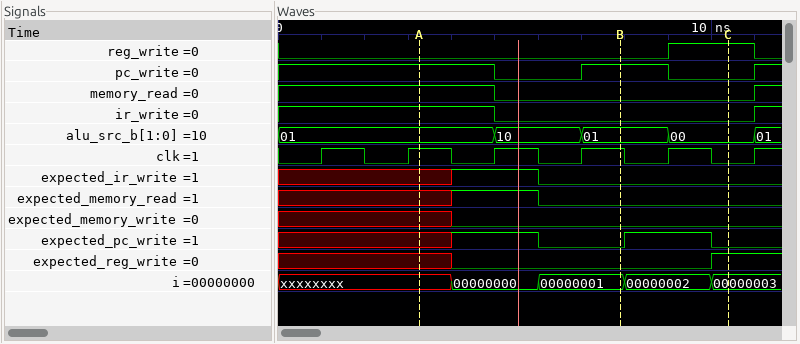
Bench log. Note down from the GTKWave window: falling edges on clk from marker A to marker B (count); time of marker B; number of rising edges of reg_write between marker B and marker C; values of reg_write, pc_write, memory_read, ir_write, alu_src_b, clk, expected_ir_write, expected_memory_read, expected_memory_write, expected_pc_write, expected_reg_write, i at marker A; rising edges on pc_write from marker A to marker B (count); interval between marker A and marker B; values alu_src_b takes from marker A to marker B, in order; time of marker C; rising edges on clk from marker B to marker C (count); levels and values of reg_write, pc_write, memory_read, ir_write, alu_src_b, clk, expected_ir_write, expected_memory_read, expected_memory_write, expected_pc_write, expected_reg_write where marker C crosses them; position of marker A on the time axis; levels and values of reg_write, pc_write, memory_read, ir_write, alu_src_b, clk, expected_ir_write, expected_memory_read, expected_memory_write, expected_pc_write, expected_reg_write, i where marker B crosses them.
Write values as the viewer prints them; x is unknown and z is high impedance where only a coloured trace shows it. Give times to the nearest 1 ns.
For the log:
2
8 ns
1
reg_write=0, pc_write=1, memory_read=1, ir_write=1, alu_src_b=01, clk=1, expected_ir_write=x, expected_memory_read=x, expected_memory_write=x, expected_pc_write=x, expected_reg_write=x, i=xxxxxxxx
1
5 ns
01, 10, 01
10 ns
1
reg_write=1, pc_write=0, memory_read=0, ir_write=0, alu_src_b=00, clk=0, expected_ir_write=0, expected_memory_read=0, expected_memory_write=0, expected_pc_write=0, expected_reg_write=1
3 ns
reg_write=0, pc_write=1, memory_read=0, ir_write=0, alu_src_b=01, clk=1, expected_ir_write=0, expected_memory_read=0, expected_memory_write=0, expected_pc_write=0, expected_reg_write=0, i=00000001
